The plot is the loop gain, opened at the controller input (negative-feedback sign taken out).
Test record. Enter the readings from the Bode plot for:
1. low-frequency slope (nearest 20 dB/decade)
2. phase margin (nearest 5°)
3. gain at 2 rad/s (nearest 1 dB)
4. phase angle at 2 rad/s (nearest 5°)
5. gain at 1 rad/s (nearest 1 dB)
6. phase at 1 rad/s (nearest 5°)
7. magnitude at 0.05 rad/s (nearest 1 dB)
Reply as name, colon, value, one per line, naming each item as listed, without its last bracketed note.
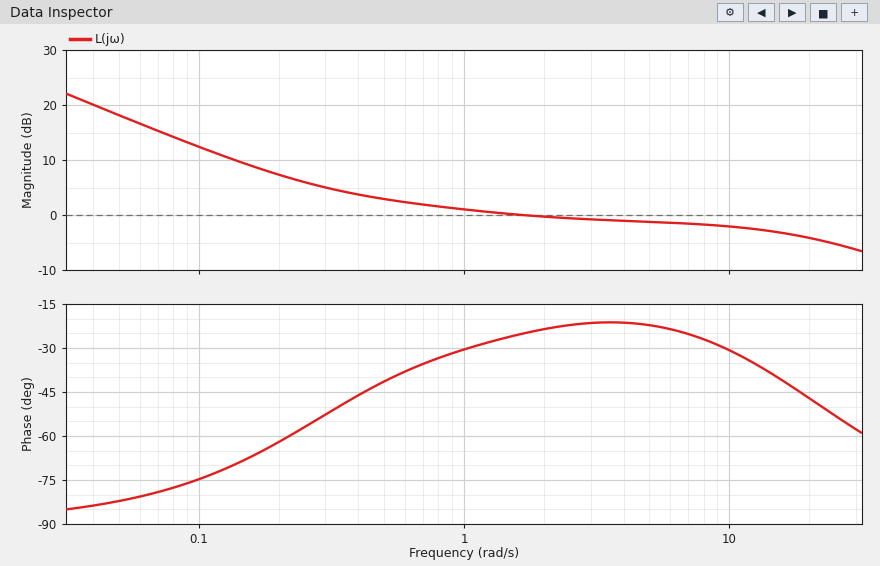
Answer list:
low-frequency slope: -20 dB/decade
phase margin: 155°
gain at 2 rad/s: 0 dB
phase angle at 2 rad/s: -25°
gain at 1 rad/s: 1 dB
phase at 1 rad/s: -30°
magnitude at 0.05 rad/s: 18 dB
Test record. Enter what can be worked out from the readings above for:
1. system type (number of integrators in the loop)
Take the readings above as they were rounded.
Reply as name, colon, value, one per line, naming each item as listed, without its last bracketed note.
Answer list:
system type: 1
